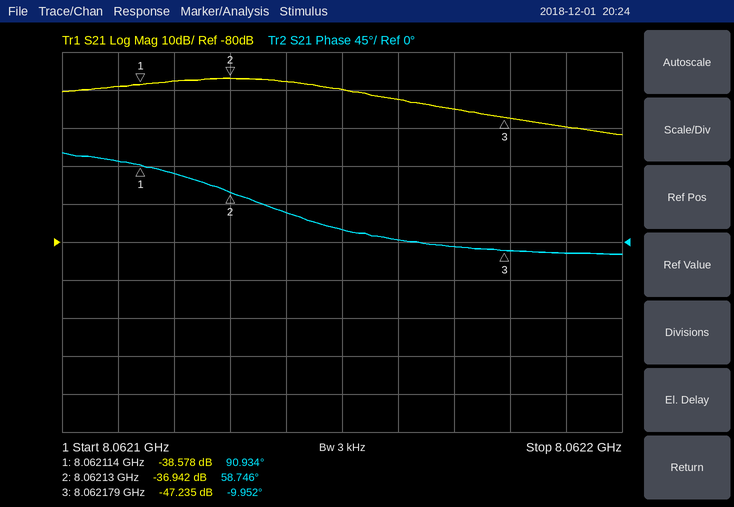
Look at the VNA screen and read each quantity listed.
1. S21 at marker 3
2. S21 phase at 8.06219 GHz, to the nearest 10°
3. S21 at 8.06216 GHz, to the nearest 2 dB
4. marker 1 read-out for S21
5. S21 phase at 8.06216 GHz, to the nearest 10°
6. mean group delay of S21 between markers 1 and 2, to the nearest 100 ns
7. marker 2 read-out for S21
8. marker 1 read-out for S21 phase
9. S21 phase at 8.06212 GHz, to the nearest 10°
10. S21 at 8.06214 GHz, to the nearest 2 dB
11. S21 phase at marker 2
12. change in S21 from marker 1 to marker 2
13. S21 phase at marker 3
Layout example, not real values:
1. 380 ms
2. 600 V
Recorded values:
1. -47.235 dB
2. -10°
3. -42 dB
4. -38.578 dB
5. 0°
6. 5.6 µs
7. -36.942 dB
8. 90.934°
9. 80°
10. -38 dB
11. 58.746°
12. 1.636 dB
13. -9.952°
